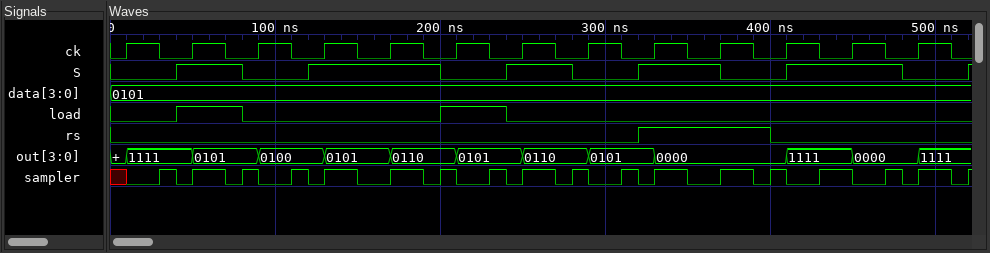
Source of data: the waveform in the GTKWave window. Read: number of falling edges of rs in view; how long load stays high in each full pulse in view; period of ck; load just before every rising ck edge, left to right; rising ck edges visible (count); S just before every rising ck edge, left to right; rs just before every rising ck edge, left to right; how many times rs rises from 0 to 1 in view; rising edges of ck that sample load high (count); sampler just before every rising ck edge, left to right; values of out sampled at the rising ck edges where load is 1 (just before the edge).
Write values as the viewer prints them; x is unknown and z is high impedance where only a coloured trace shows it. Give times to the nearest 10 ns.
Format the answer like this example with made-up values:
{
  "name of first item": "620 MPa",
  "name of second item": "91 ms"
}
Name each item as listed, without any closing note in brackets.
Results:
{
  "number of falling edges of rs in view": "1",
  "how long load stays high in each full pulse in view": "40 ns, 40 ns",
  "period of ck": "40 ns",
  "load just before every rising ck edge, left to right": "0 1 0 0 0 1 0 0 0 0 0 0 0",
  "rising ck edges visible": "13",
  "S just before every rising ck edge, left to right": "0 1 0 1 1 0 1 0 1 1 0 1 0",
  "rs just before every rising ck edge, left to right": "0 0 0 0 0 0 0 0 1 1 0 0 0",
  "how many times rs rises from 0 to 1 in view": "1",
  "rising edges of ck that sample load high": "2",
  "sampler just before every rising ck edge, left to right": "x 0 1 0 0 1 0 1 0 0 1 1 0",
  "values of out sampled at the rising ck edges where load is 1": "1111, 0110"
}
